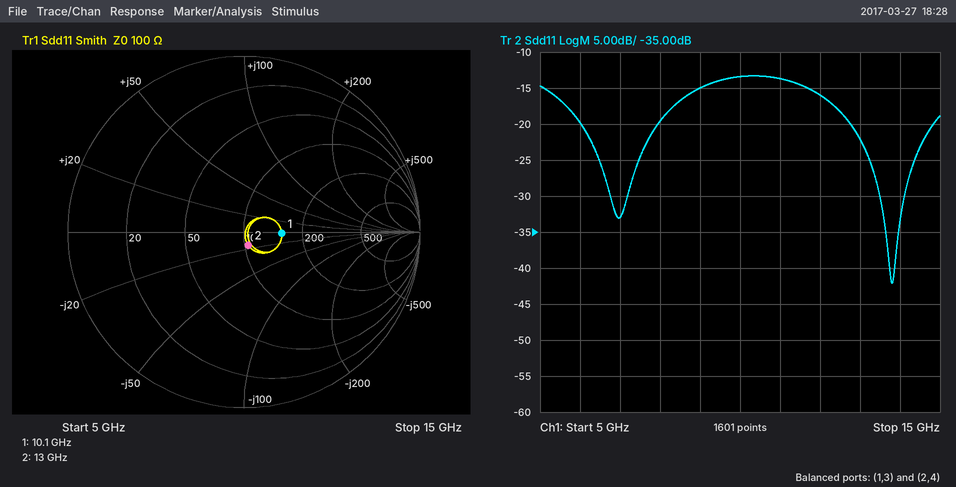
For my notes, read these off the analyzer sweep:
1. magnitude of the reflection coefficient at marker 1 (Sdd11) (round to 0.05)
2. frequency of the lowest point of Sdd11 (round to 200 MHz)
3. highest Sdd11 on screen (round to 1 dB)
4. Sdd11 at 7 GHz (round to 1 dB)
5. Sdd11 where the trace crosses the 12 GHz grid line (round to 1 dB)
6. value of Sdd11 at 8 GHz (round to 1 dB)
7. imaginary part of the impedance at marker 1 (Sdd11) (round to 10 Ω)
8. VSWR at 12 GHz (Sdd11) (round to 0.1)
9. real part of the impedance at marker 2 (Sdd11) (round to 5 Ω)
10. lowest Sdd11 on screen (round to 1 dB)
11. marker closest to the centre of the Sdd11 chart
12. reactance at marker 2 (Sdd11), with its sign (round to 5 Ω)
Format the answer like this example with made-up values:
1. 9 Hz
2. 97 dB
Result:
1. 0.20
2. 13.8 GHz
3. -13 dB
4. -33 dB
5. -16 dB
6. -20 dB
7. 0 Ω
8. 1.4
9. 105 Ω
10. -42 dB
11. marker 2
12. -15 Ω
